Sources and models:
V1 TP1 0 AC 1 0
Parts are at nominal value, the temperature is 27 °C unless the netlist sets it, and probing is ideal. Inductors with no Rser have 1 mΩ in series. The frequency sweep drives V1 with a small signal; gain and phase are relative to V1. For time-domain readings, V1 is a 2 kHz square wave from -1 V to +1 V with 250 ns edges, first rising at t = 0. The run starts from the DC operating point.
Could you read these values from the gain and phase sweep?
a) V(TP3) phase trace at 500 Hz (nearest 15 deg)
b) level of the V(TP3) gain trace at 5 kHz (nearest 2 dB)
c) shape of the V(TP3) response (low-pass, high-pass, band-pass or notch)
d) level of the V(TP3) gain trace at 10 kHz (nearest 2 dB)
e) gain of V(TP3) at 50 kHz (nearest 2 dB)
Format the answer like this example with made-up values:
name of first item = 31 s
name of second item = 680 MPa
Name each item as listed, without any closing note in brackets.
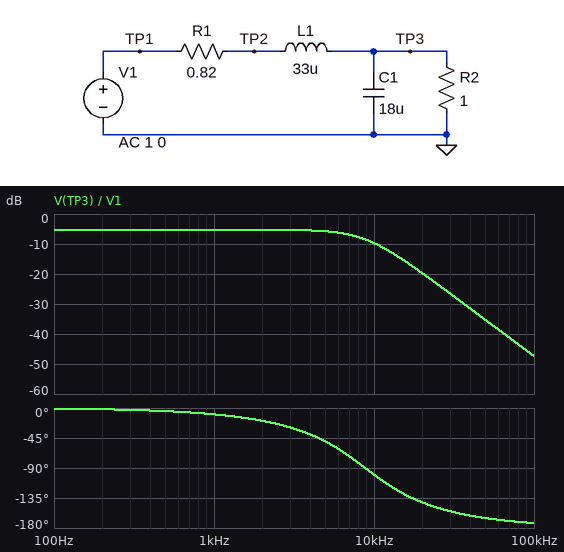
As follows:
V(TP3) phase trace at 500 Hz = 0 deg
level of the V(TP3) gain trace at 5 kHz = -6 dB
shape of the V(TP3) response = low-pass
level of the V(TP3) gain trace at 10 kHz = -10 dB
gain of V(TP3) at 50 kHz = -36 dB
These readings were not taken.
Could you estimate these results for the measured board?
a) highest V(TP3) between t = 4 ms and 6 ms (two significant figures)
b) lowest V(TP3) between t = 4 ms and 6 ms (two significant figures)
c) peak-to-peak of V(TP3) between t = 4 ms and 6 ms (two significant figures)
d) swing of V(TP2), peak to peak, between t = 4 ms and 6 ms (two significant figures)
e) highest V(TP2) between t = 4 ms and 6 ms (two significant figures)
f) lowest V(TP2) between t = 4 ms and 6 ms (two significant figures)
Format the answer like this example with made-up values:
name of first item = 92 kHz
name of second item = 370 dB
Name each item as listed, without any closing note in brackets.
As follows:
highest V(TP3) between t = 4 ms and 6 ms = 590 mV
lowest V(TP3) between t = 4 ms and 6 ms = -590 mV
peak-to-peak of V(TP3) between t = 4 ms and 6 ms = 1.2 V
swing of V(TP2), peak to peak, between t = 4 ms and 6 ms = 2.9 V
highest V(TP2) between t = 4 ms and 6 ms = 1.4 V
lowest V(TP2) between t = 4 ms and 6 ms = -1.4 V
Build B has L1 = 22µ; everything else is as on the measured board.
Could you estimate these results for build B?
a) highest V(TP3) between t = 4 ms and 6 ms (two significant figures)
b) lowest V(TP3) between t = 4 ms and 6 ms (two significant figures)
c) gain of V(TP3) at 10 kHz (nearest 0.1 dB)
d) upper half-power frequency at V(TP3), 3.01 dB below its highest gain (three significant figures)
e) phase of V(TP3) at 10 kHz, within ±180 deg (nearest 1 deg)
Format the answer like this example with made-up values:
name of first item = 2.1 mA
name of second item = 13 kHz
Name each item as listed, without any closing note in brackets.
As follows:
highest V(TP3) between t = 4 ms and 6 ms = 610 mV
lowest V(TP3) between t = 4 ms and 6 ms = -610 mV
gain of V(TP3) at 10 kHz = -7.3 dB
upper half-power frequency at V(TP3), 3.01 dB below its highest gain = 11.1 kHz
phase of V(TP3) at 10 kHz, within ±180 deg = -84 deg
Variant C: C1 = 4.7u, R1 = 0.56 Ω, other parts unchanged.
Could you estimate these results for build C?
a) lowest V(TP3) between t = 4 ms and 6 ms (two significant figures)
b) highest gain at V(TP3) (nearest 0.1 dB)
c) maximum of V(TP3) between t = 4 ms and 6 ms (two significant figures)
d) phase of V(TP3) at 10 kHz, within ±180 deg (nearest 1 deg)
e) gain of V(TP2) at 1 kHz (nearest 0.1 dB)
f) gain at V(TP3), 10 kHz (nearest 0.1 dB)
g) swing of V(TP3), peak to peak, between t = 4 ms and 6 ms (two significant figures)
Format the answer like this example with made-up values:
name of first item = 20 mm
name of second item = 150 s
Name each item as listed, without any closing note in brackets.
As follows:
lowest V(TP3) between t = 4 ms and 6 ms = -640 mV
highest gain at V(TP3) = -3.9 dB
maximum of V(TP3) between t = 4 ms and 6 ms = 640 mV
phase of V(TP3) at 10 kHz, within ±180 deg = -67 deg
gain of V(TP2) at 1 kHz = -3.8 dB
gain at V(TP3), 10 kHz = -7.7 dB
swing of V(TP3), peak to peak, between t = 4 ms and 6 ms = 1.3 V
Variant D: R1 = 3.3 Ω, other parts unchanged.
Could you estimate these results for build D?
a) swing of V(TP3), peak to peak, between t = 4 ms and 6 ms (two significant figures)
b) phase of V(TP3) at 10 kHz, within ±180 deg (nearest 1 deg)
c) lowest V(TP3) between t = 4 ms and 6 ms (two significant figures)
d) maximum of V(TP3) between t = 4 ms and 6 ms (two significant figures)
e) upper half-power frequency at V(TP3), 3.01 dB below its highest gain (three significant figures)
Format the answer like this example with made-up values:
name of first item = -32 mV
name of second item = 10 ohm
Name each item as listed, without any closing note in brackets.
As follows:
swing of V(TP3), peak to peak, between t = 4 ms and 6 ms = 470 mV
phase of V(TP3) at 10 kHz, within ±180 deg = -71 deg
lowest V(TP3) between t = 4 ms and 6 ms = -230 mV
maximum of V(TP3) between t = 4 ms and 6 ms = 230 mV
upper half-power frequency at V(TP3), 3.01 dB below its highest gain = 9.89 kHz
